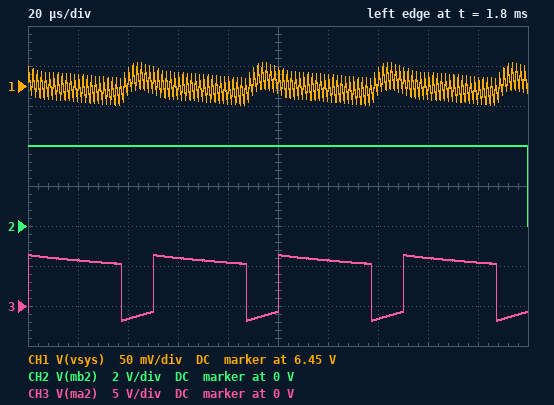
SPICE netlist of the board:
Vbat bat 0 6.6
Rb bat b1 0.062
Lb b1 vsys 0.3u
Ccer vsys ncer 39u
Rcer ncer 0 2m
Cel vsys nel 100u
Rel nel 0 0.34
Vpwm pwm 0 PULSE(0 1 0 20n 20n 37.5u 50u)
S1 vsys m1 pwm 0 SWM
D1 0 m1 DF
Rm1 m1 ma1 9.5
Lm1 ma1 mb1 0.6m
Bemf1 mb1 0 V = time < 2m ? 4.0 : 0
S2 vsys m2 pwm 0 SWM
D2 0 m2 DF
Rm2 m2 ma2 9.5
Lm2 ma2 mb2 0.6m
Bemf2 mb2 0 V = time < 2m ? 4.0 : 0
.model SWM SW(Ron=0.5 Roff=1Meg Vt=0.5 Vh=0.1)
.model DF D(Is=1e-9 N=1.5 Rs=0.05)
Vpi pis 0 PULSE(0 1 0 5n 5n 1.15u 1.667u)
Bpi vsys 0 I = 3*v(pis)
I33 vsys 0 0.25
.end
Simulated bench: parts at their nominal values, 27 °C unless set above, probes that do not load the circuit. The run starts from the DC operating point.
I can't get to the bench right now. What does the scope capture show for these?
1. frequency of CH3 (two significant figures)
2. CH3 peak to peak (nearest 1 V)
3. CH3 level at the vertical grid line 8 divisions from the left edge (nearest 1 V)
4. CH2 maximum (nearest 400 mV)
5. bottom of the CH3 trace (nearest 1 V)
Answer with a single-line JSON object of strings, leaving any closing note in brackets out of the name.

{"frequency of CH3": "20 kHz", "CH3 peak to peak": "8 V", "CH3 level at the vertical grid line 8 divisions from the left edge": "6 V", "CH2 maximum": "4.0 V", "bottom of the CH3 trace": "-2 V"}
